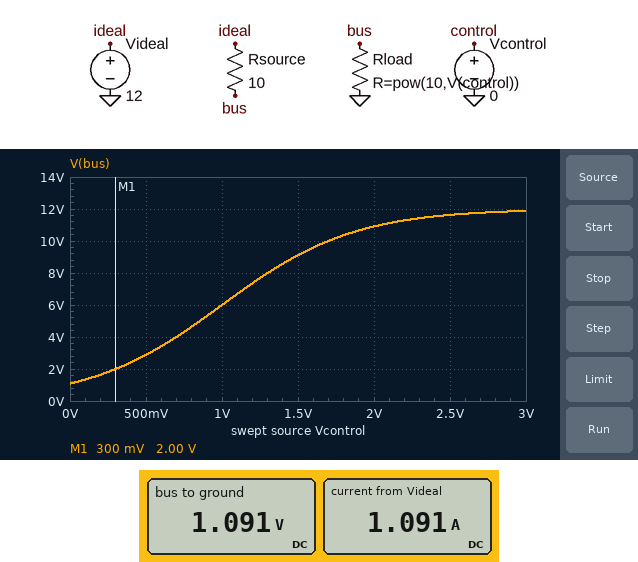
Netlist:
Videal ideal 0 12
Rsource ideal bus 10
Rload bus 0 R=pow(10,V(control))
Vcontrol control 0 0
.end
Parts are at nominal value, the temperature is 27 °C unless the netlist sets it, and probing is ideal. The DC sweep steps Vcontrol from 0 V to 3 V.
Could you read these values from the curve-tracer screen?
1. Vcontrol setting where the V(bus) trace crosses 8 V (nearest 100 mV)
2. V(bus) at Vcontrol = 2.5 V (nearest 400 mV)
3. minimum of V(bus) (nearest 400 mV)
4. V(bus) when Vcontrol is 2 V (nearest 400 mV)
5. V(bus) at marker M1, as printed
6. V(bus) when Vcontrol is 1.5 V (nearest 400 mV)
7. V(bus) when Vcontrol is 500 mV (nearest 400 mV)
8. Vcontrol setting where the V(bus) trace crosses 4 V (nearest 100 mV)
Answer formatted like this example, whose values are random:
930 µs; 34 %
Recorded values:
1.3 V; 11.6 V; 1.2 V; 10.8 V; 2.00 V; 9.2 V; 2.8 V; 700 mV
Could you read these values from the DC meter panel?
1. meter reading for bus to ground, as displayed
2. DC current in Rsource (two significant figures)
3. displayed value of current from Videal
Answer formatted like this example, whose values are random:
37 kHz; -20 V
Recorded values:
1.091 V; 1.1 A; 1.091 A
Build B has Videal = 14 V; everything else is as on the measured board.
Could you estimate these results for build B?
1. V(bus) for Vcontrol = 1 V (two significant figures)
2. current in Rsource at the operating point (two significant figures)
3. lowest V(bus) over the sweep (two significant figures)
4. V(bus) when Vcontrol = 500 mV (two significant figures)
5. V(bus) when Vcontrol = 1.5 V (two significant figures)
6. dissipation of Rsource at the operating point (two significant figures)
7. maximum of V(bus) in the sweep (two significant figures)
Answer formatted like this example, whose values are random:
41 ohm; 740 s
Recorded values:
7.0 V; 1.3 A; 1.3 V; 3.4 V; 11 V; 16 W; 14 V
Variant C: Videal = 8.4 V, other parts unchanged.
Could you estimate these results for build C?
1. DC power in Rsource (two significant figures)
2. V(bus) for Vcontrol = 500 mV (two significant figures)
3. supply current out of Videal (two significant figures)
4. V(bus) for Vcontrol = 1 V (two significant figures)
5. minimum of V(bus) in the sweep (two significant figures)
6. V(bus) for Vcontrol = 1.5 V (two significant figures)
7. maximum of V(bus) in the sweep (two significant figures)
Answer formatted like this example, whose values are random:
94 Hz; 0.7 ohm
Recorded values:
5.8 W; 2.0 V; 760 mA; 4.2 V; 760 mV; 6.4 V; 8.3 V
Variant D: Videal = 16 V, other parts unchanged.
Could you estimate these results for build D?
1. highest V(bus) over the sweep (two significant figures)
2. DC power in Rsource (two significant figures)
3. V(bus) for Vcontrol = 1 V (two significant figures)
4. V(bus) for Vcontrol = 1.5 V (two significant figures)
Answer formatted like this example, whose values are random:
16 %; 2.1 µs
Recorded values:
16 V; 21 W; 8.0 V; 12 V
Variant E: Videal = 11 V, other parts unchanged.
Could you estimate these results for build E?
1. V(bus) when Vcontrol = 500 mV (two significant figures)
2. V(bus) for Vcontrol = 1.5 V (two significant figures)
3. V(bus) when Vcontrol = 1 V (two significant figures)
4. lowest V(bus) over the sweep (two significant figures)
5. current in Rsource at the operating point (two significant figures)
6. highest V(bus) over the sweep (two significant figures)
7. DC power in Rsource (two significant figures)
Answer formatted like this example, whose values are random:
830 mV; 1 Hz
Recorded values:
2.6 V; 8.4 V; 5.5 V; 1.0 V; 1.0 A; 11 V; 10 W
